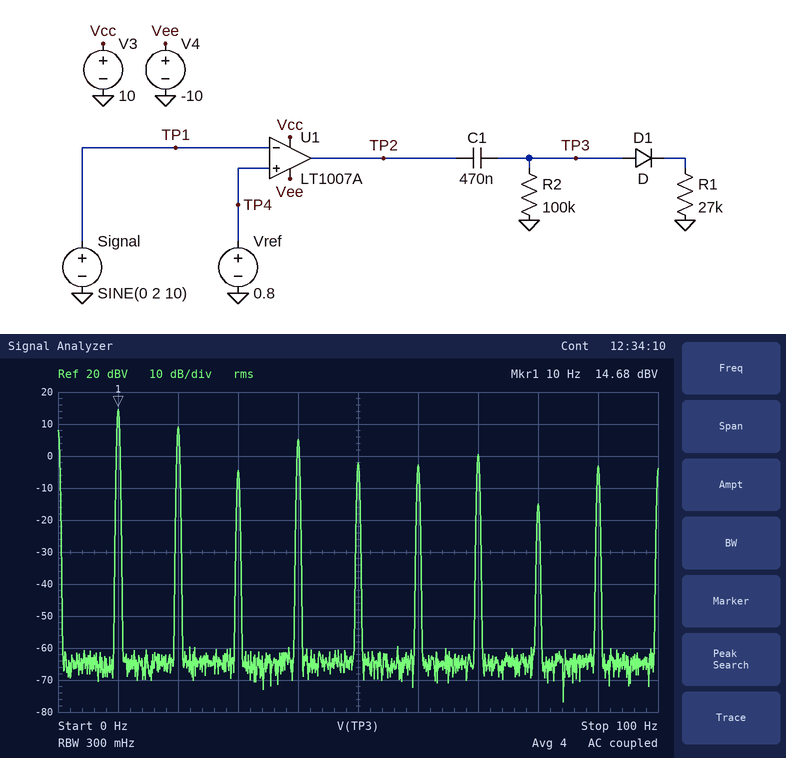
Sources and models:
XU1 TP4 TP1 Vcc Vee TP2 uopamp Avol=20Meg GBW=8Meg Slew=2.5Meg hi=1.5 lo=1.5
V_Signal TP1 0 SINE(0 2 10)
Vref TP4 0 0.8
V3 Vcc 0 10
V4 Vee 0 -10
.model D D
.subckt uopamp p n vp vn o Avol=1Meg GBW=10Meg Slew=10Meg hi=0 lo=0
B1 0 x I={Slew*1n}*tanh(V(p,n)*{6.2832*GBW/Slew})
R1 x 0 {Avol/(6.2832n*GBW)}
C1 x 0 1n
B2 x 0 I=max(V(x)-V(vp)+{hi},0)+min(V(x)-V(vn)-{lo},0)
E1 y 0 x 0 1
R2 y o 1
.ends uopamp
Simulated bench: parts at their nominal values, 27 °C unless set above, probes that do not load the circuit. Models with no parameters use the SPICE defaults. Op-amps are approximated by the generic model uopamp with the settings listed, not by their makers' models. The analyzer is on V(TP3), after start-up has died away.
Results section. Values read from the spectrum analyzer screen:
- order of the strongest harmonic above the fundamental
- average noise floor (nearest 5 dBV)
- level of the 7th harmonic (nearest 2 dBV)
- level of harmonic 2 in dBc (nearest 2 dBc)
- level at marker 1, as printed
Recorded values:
2
-65 dBV
0 dBV
-6 dBc
14.68 dBV
